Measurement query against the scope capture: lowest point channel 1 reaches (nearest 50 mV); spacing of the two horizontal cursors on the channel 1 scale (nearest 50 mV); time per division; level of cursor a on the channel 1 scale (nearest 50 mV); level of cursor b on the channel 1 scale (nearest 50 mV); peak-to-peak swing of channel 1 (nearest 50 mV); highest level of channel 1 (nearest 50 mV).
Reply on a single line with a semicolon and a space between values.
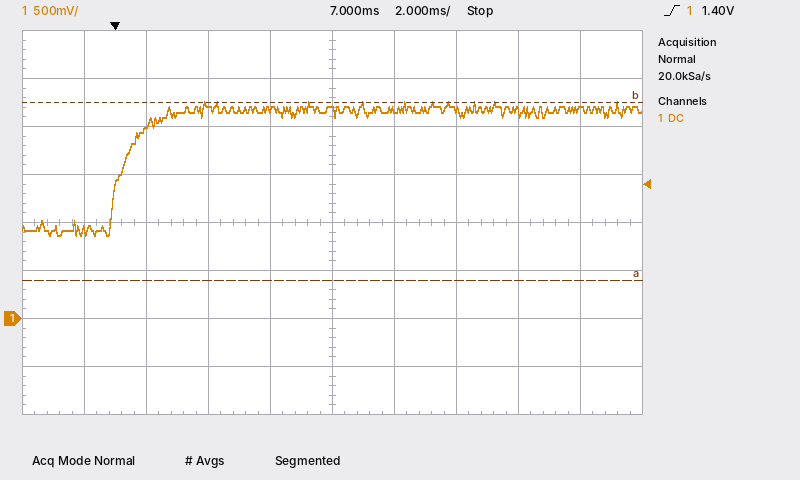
850 mV; 1.85 V; 2 ms; 400 mV; 2.25 V; 1.40 V; 2.25 V
